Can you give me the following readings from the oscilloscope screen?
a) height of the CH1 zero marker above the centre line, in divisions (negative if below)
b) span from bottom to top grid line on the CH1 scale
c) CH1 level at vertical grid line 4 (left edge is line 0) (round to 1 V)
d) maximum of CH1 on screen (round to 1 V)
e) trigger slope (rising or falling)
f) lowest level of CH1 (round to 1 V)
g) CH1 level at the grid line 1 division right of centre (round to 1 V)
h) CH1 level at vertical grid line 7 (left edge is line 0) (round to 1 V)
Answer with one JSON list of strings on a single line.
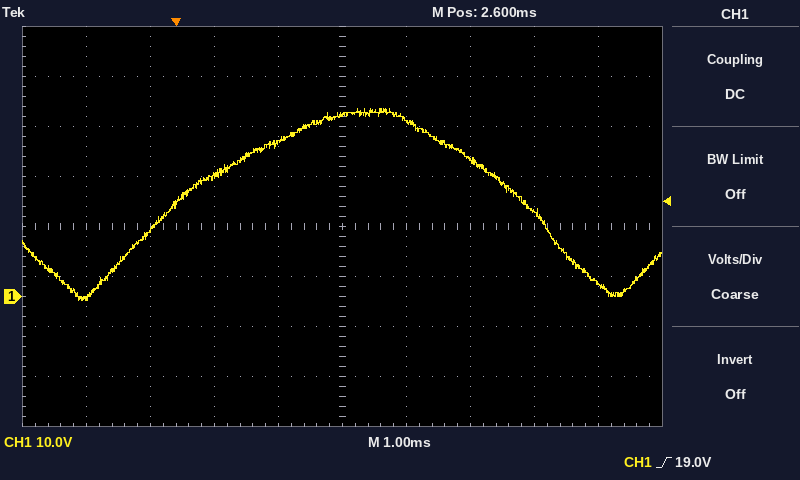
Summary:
["-1.4 div", "80 V", "31 V", "38 V", "rising", "-1 V", "35 V", "27 V"]
